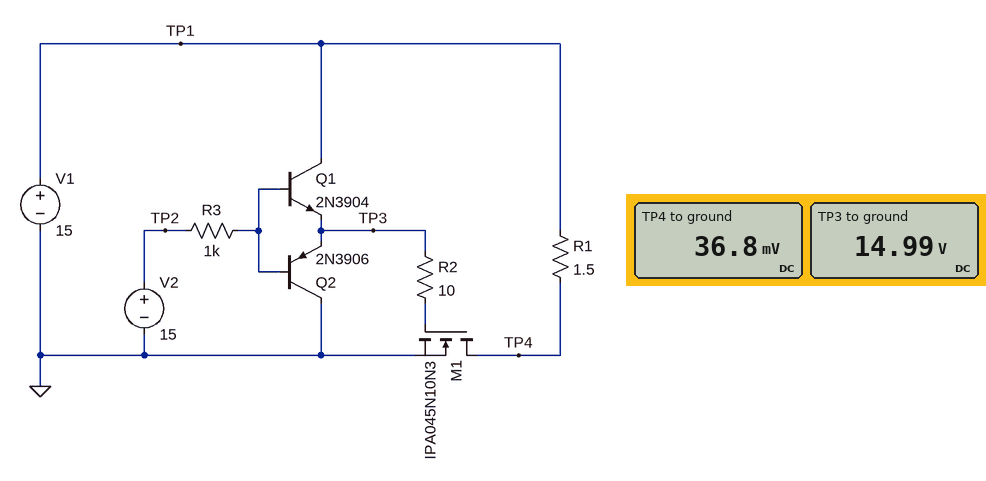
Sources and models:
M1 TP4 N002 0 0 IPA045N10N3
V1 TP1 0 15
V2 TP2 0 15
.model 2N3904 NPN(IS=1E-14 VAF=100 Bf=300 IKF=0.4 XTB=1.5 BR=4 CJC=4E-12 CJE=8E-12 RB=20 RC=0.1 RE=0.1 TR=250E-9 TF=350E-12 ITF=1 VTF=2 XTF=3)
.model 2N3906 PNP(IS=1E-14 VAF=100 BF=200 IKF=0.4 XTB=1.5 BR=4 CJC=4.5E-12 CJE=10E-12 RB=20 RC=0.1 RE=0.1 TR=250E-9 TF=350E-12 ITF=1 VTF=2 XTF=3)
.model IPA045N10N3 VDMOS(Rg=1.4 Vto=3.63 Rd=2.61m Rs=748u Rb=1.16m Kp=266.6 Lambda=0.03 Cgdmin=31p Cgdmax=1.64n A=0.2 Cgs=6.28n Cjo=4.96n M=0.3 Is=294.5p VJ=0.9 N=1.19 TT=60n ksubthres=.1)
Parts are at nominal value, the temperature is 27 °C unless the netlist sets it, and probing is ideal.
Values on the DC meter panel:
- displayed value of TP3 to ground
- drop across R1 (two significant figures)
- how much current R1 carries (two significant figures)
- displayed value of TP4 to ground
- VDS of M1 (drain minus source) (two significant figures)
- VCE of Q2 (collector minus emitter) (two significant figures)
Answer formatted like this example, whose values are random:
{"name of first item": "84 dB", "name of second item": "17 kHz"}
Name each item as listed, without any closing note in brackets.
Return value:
{"displayed value of TP3 to ground": "14.99 V", "drop across R1": "15 V", "how much current R1 carries": "10 A", "displayed value of TP4 to ground": "36.8 mV", "VDS of M1 (drain minus source)": "37 mV", "VCE of Q2 (collector minus emitter)": "-15 V"}
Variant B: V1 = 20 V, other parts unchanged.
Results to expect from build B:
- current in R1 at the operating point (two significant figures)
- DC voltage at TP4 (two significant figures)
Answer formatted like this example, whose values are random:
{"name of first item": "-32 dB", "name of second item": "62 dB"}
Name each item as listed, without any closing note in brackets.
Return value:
{"current in R1 at the operating point": "13 A", "DC voltage at TP4": "49 mV"}
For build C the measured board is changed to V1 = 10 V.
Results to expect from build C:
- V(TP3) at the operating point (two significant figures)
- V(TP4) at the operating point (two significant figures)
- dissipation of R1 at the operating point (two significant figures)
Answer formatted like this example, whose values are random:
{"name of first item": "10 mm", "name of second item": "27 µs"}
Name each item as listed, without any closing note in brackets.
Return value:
{"V(TP3) at the operating point": "10 V", "V(TP4) at the operating point": "26 mV", "dissipation of R1 at the operating point": "66 W"}
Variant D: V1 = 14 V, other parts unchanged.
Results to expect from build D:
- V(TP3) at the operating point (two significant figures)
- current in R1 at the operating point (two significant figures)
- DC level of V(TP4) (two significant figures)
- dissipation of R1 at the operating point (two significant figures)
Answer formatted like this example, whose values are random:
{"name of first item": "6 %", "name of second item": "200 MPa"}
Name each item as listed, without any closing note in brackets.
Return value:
{"V(TP3) at the operating point": "14 V", "current in R1 at the operating point": "9.3 A", "DC level of V(TP4)": "35 mV", "dissipation of R1 at the operating point": "130 W"}
